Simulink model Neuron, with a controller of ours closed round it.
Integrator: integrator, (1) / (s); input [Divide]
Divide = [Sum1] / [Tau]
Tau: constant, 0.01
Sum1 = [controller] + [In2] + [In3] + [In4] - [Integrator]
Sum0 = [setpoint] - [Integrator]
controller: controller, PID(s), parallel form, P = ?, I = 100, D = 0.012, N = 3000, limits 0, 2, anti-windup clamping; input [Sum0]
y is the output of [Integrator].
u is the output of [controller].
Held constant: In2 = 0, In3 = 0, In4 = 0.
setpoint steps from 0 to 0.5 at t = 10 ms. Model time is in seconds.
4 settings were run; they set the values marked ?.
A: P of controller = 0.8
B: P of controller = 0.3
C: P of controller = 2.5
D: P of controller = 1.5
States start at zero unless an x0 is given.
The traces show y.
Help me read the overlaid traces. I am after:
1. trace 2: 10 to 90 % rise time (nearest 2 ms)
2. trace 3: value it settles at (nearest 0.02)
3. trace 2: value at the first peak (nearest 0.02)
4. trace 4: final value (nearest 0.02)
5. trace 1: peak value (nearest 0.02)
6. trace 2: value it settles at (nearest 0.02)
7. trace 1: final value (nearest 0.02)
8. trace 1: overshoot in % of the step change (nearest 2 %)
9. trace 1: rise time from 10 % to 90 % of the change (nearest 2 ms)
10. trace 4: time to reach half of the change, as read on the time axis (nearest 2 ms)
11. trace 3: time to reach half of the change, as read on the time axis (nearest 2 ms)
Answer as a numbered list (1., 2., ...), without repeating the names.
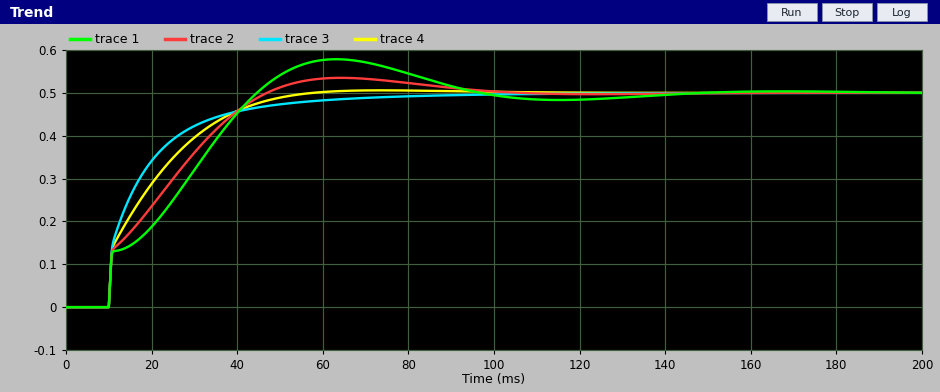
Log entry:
1. 28 ms
2. 0.50
3. 0.54
4. 0.50
5. 0.58
6. 0.50
7. 0.50
8. 16 %
9. 30 ms
10. 18 ms
11. 14 ms
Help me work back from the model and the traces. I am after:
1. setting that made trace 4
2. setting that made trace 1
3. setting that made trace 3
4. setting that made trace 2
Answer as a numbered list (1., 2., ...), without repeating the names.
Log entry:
1. D
2. B
3. C
4. A
